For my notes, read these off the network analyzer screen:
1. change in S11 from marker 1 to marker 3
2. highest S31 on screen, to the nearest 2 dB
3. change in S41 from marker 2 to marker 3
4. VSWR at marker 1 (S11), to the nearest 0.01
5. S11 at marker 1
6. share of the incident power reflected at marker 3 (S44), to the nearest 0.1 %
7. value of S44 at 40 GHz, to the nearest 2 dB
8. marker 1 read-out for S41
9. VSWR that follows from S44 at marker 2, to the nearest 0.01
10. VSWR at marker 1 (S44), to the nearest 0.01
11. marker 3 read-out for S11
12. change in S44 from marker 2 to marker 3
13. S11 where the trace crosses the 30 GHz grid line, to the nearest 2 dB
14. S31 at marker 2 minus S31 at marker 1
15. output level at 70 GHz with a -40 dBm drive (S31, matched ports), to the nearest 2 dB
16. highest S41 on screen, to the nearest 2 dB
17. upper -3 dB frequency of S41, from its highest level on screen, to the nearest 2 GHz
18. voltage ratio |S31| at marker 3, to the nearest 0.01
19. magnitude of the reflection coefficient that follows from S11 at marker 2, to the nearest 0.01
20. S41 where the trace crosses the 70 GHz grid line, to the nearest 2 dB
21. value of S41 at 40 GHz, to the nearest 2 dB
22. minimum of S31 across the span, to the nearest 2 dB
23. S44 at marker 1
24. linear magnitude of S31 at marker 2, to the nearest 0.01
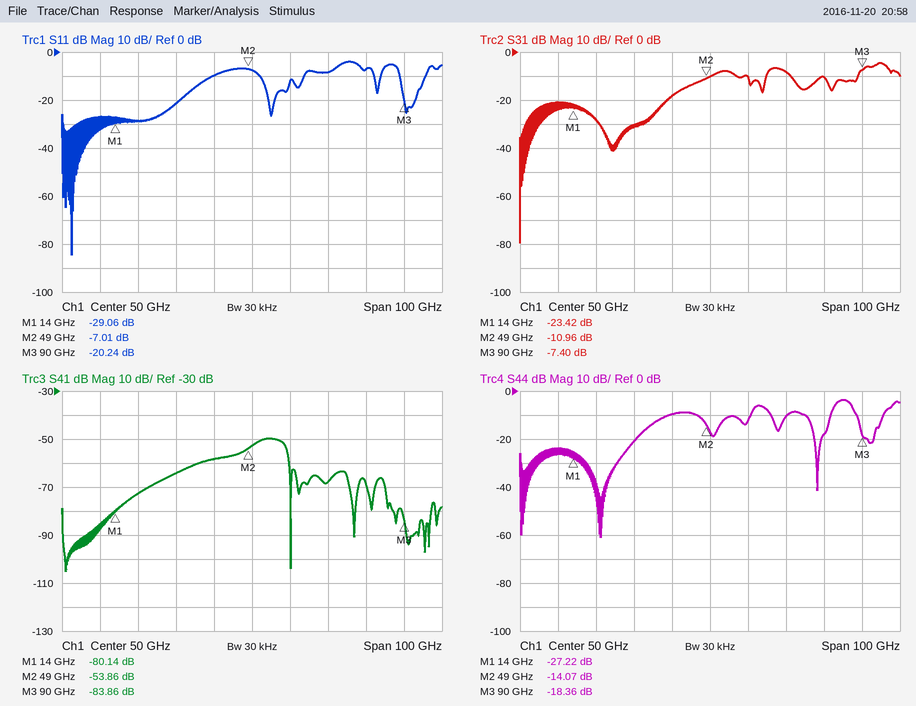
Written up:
8.82 dB
-4 dB
-30.00 dB
1.07
-29.06 dB
1.5 %
-10 dB
-80.14 dB
1.49
1.09
-20.24 dB
-4.29 dB
-22 dB
12.46 dB
-48 dBm
-50 dB
58 GHz
0.43
0.45
-68 dB
-58 dB
-80 dB
-27.22 dB
0.28
